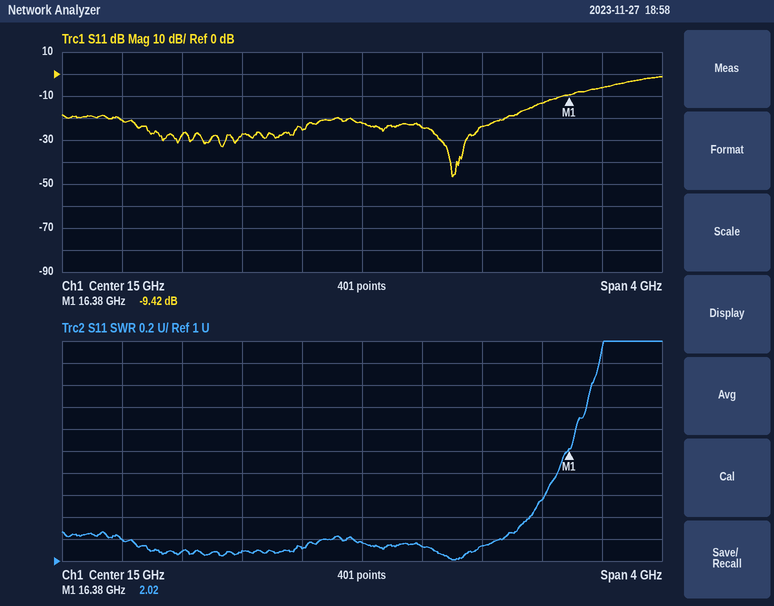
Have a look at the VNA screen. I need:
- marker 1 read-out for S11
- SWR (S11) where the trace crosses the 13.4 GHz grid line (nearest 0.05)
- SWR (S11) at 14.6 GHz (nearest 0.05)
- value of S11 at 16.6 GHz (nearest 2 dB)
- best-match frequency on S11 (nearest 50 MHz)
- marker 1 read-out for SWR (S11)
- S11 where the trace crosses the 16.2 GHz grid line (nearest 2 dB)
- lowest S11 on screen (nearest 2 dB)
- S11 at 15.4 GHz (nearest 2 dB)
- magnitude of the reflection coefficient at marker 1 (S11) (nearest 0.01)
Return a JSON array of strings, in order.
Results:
["-9.42 dB", "1.20", "1.10", "-6 dB", "15.60 GHz", "2.02", "-14 dB", "-46 dB", "-24 dB", "0.34"]
